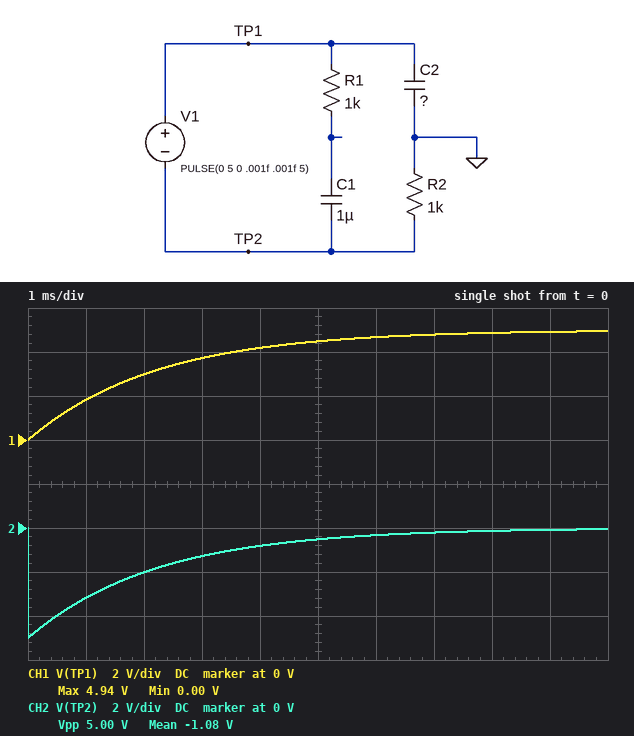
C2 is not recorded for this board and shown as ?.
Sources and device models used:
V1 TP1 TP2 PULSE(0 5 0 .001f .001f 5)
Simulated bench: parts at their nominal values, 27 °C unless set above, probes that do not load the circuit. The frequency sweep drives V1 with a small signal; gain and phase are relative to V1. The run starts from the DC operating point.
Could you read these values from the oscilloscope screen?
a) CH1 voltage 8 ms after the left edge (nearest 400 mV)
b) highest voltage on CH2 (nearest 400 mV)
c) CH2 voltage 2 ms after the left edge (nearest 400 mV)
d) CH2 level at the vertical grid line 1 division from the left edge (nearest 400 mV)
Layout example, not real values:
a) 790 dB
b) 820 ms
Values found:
a) 4.8 V
b) 0 V
c) -2.0 V
d) -3.2 V
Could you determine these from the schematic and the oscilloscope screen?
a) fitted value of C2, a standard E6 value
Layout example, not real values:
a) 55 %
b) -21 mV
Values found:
a) 2.2 µF
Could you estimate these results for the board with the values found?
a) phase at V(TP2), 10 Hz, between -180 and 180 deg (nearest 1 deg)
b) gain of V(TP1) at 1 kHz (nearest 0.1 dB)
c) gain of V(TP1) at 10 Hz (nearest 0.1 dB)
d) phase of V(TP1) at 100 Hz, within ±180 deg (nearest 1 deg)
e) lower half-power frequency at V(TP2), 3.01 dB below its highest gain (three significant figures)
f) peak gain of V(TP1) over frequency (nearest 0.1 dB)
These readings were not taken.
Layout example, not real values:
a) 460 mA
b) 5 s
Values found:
a) -98 deg
b) -22.8 dB
c) -0.1 dB
d) -54 deg
e) 72.3 Hz
f) 0 dB
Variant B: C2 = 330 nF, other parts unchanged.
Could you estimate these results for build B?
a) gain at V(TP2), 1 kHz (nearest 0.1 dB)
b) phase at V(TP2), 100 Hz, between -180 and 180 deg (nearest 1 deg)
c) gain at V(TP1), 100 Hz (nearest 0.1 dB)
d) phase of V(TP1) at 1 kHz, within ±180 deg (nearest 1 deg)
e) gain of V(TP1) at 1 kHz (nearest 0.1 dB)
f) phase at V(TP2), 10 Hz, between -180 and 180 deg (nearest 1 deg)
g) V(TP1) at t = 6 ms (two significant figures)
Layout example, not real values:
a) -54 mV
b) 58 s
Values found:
a) -0.9 dB
b) -102 deg
c) -0.2 dB
d) -64 deg
e) -7.2 dB
f) -91 deg
g) 5.0 V
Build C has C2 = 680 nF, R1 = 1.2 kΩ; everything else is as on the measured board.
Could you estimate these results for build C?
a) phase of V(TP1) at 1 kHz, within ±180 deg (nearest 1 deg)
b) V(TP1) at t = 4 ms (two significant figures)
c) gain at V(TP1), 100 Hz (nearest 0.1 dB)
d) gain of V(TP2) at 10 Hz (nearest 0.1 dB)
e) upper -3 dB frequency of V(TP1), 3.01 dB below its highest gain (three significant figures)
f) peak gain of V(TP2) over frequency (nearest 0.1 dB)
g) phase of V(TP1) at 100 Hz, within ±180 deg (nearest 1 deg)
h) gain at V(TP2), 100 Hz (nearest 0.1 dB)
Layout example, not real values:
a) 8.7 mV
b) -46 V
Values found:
a) -77 deg
b) 5.0 V
c) -0.7 dB
d) -27.4 dB
e) 234 Hz
f) 0 dB
g) -23 deg
h) -8.1 dB
